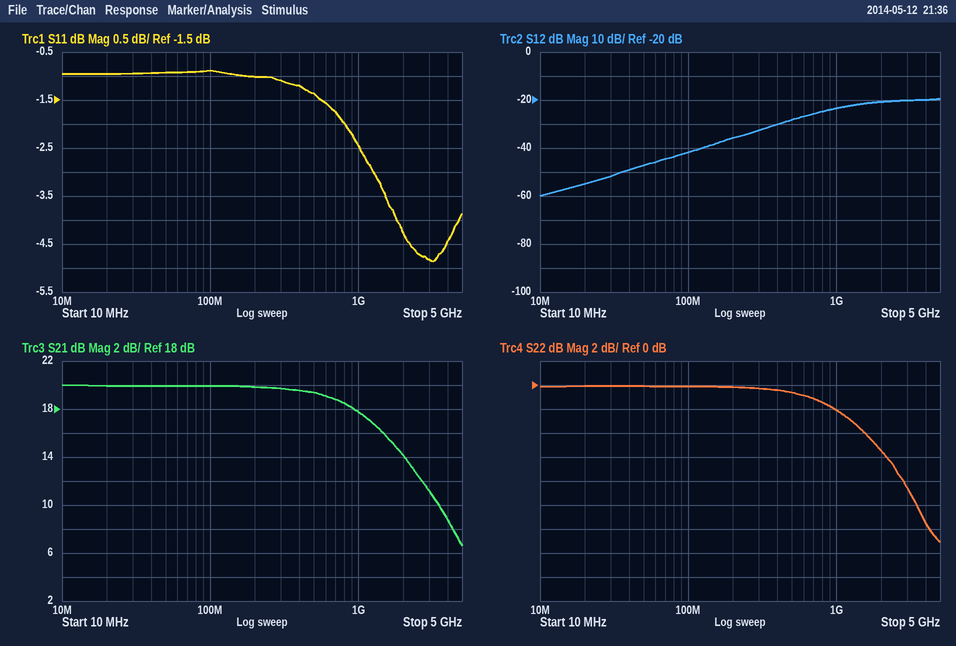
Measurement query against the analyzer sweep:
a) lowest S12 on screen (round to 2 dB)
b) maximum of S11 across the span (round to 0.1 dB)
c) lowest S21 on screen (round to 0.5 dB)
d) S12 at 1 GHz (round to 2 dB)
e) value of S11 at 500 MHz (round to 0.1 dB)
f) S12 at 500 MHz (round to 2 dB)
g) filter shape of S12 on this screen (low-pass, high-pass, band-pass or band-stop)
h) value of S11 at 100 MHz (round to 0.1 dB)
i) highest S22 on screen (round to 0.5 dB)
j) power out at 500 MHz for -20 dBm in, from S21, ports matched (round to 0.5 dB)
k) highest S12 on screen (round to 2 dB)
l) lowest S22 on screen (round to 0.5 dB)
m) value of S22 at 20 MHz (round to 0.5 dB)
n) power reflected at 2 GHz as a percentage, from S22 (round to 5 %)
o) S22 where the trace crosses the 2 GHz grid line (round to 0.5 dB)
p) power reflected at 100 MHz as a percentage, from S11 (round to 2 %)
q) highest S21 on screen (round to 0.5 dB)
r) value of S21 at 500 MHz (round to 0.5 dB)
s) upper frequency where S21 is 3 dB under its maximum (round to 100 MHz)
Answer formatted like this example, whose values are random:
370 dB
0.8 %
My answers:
-60 dB
-0.9 dB
6.5 dB
-24 dB
-1.4 dB
-28 dB
high-pass
-0.9 dB
0.0 dB
-0.5 dBm
-20 dB
-13.0 dB
0.0 dB
30 %
-5.5 dB
82 %
20.0 dB
19.5 dB
1.2 GHz
